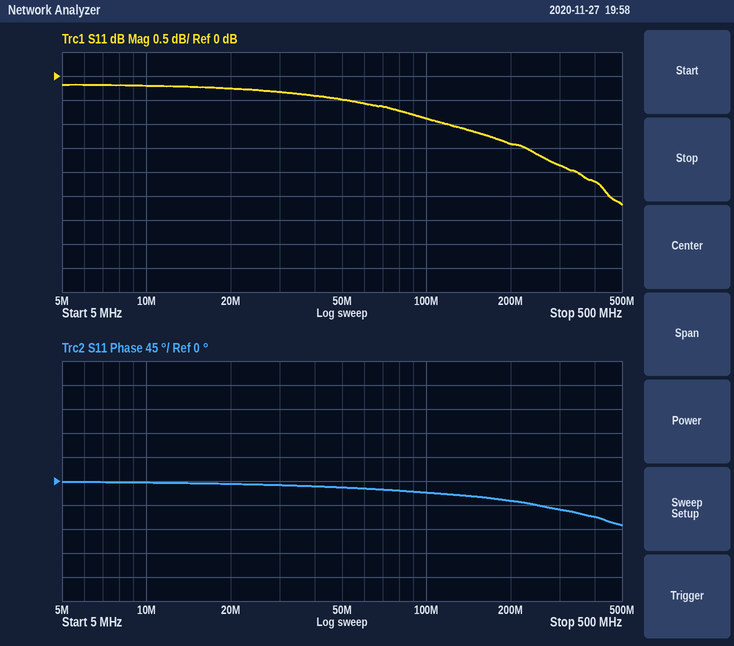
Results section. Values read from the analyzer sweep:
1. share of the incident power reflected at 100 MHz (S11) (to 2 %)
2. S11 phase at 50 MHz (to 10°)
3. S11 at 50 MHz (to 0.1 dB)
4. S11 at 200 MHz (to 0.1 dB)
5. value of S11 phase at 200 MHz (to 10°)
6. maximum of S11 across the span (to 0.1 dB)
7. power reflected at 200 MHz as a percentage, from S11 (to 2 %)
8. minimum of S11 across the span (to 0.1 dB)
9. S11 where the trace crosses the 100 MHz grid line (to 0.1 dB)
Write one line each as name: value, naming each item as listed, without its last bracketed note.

share of the incident power reflected at 100 MHz (S11): 82 %
S11 phase at 50 MHz: -10°
S11 at 50 MHz: -0.5 dB
S11 at 200 MHz: -1.4 dB
value of S11 phase at 200 MHz: -40°
maximum of S11 across the span: -0.2 dB
power reflected at 200 MHz as a percentage, from S11: 72 %
minimum of S11 across the span: -2.7 dB
S11 where the trace crosses the 100 MHz grid line: -0.9 dB
